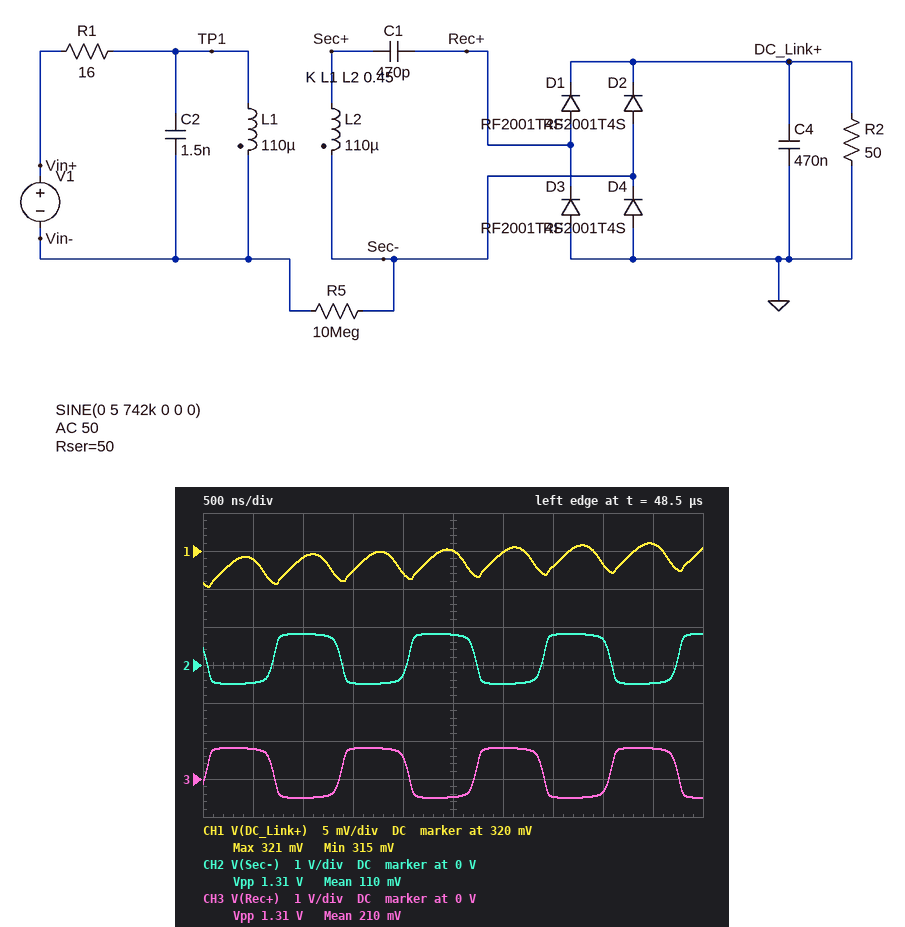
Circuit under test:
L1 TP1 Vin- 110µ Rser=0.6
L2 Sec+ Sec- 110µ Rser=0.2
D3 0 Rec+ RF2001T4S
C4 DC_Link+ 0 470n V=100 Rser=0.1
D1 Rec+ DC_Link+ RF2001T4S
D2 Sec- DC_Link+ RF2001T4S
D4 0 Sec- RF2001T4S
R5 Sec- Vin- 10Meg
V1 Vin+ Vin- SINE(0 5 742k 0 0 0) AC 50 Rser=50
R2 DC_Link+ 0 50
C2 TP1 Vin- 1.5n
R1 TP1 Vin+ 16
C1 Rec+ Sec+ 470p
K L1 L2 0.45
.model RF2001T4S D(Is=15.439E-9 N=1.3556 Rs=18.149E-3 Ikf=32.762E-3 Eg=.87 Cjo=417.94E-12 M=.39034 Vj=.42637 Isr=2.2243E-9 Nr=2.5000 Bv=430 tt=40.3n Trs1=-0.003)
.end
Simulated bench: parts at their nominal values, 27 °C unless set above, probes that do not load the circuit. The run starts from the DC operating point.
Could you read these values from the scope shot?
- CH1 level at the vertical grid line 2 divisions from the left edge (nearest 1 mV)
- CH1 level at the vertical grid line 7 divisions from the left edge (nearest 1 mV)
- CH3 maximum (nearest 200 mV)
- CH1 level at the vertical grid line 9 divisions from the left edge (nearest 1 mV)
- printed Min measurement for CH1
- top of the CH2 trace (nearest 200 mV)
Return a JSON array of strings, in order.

["319 mV", "318 mV", "800 mV", "321 mV", "315 mV", "800 mV"]
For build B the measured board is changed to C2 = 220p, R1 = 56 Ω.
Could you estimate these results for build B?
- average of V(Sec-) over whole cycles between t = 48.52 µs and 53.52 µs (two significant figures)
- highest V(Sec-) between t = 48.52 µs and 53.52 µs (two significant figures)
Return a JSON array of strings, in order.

["170 mV", "840 mV"]
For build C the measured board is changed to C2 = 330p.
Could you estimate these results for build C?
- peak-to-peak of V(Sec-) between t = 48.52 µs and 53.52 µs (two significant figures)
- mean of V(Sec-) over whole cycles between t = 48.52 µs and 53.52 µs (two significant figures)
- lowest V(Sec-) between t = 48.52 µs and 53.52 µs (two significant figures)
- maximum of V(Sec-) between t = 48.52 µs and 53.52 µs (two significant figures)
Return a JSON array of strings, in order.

["1.4 V", "180 mV", "-500 mV", "870 mV"]
